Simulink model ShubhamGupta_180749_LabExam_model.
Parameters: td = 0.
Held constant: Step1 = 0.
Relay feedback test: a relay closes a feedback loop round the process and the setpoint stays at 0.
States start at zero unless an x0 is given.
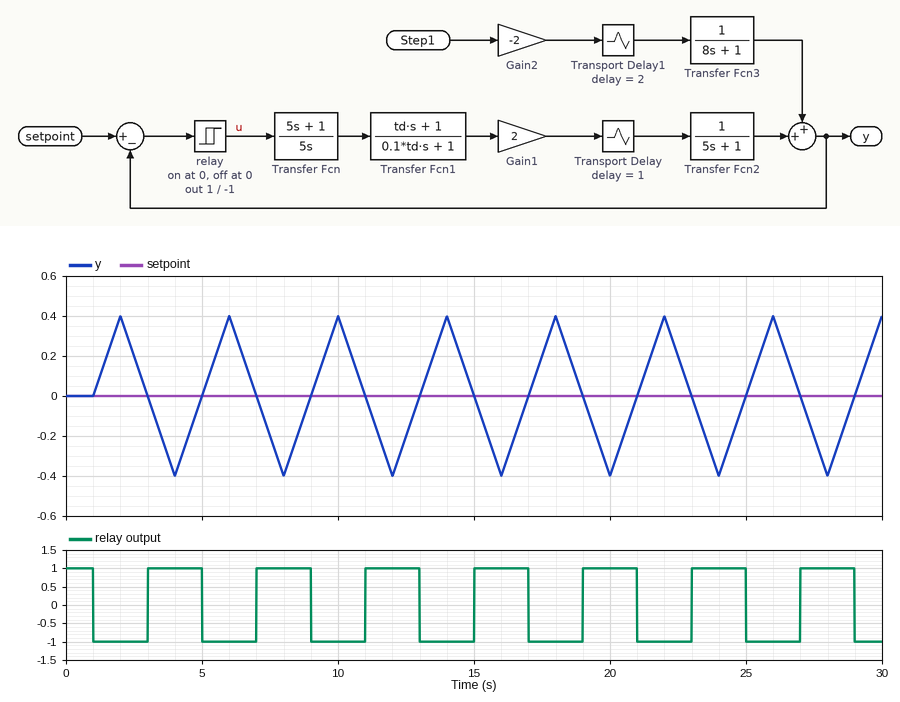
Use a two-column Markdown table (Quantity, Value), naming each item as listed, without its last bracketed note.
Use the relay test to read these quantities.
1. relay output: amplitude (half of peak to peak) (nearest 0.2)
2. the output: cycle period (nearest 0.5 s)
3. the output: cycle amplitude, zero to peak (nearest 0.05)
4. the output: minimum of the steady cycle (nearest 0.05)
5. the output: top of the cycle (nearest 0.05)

| Quantity | Value |
|---|---|
| relay output: amplitude (half of peak to peak) | 1.0 |
| the output: cycle period | 4.0 s |
| the output: cycle amplitude, zero to peak | 0.40 |
| the output: minimum of the steady cycle | -0.40 |
| the output: top of the cycle | 0.40 |
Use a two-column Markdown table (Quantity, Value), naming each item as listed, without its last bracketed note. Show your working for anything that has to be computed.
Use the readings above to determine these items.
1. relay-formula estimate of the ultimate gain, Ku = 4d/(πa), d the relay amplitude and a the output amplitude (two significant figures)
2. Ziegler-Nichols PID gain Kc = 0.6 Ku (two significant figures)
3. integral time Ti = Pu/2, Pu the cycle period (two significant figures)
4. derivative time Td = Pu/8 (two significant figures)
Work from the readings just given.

| Quantity | Value |
|---|---|
| relay-formula estimate of the ultimate gain, Ku = 4d/(πa), d the relay amplitude and a the output amplitude | 4 × 1 / (π × 0.4) = 3.2 |
| Ziegler-Nichols PID gain Kc = 0.6 Ku | 0.6 × 3.2 = 1.9 |
| integral time Ti = Pu/2, Pu the cycle period | 4 / 2 = 2.0 s |
| derivative time Td = Pu/8 | 4 / 8 = 0.50 s |
